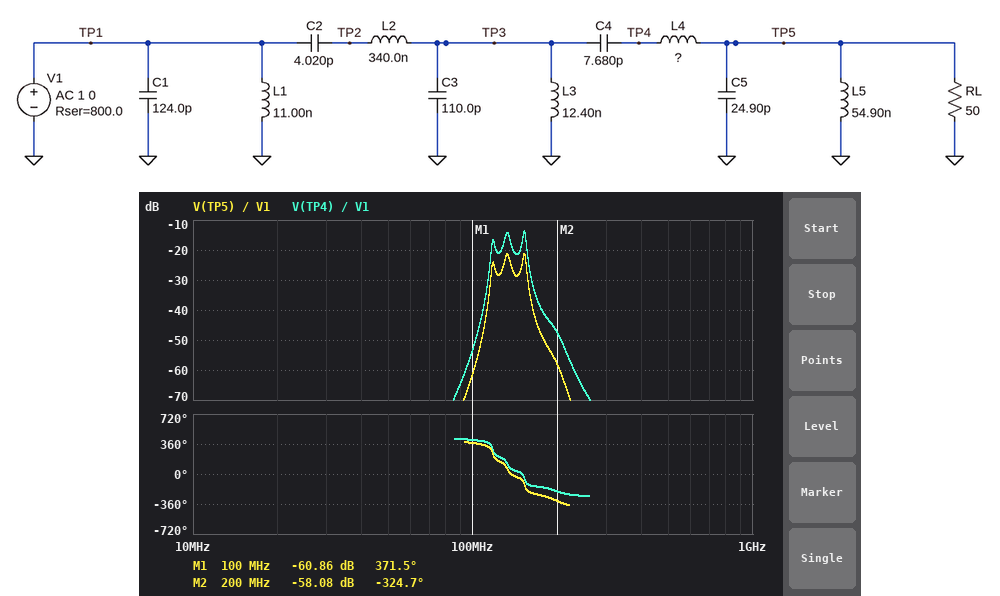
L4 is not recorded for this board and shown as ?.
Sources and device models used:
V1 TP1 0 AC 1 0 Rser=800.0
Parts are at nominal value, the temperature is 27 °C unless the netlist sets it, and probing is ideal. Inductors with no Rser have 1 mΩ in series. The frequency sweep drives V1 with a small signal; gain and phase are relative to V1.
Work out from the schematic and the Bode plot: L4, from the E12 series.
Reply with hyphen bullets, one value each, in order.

- 120 nH
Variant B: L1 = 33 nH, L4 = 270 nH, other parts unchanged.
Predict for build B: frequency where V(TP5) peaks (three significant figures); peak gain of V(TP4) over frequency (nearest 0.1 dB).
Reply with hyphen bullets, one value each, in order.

- 129 MHz
- -16.3 dB
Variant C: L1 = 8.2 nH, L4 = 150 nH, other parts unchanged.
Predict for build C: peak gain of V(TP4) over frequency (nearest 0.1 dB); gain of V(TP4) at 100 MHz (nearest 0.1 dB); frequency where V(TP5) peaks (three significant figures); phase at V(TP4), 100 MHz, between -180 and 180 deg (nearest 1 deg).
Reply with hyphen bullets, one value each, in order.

- -8.4 dB
- -54.9 dB
- 165 MHz
- 47 deg
